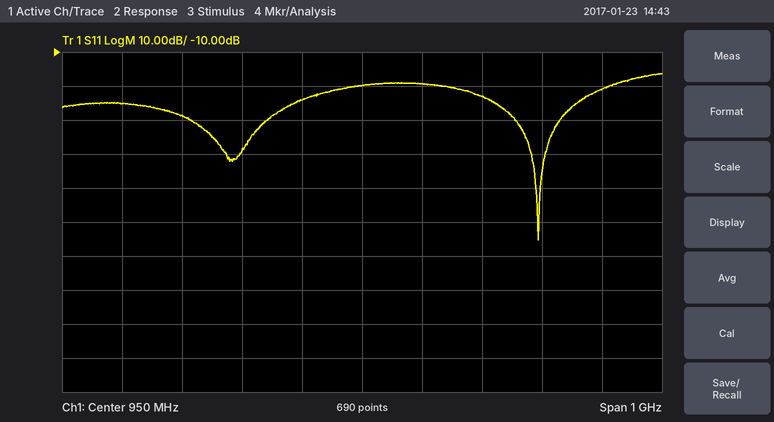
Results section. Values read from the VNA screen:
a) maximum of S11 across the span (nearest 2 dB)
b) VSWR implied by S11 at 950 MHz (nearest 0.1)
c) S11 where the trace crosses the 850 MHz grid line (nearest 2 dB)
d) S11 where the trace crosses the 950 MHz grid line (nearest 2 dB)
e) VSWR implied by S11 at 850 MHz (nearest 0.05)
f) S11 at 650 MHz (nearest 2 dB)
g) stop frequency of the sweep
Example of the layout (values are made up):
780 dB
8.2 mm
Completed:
-16 dB
1.2
-24 dB
-20 dB
1.15
-28 dB
1.45 GHz
